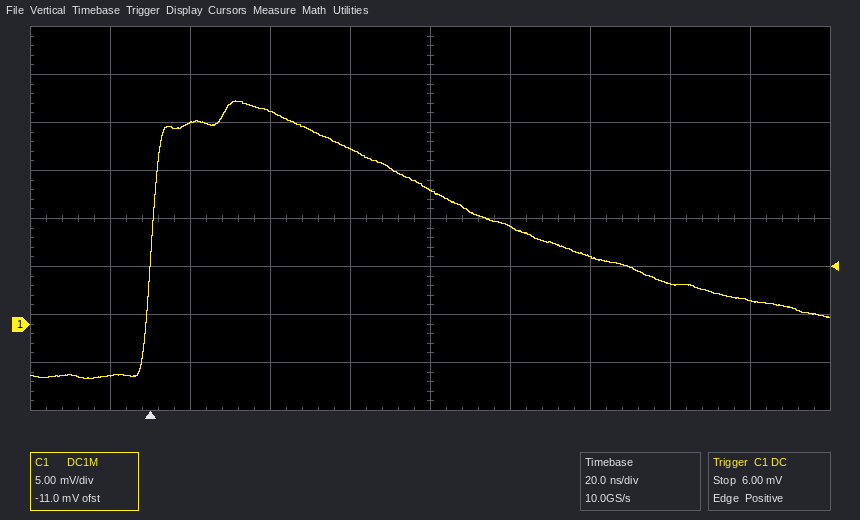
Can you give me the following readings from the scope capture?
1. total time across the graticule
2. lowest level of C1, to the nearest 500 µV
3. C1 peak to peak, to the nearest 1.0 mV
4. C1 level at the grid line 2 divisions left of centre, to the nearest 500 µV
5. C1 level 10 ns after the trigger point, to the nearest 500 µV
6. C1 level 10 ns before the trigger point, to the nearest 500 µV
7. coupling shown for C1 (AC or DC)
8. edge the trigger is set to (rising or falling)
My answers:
200 ns
-5.5 mV
29.0 mV
22.0 mV
21.0 mV
-5.5 mV
DC
rising
